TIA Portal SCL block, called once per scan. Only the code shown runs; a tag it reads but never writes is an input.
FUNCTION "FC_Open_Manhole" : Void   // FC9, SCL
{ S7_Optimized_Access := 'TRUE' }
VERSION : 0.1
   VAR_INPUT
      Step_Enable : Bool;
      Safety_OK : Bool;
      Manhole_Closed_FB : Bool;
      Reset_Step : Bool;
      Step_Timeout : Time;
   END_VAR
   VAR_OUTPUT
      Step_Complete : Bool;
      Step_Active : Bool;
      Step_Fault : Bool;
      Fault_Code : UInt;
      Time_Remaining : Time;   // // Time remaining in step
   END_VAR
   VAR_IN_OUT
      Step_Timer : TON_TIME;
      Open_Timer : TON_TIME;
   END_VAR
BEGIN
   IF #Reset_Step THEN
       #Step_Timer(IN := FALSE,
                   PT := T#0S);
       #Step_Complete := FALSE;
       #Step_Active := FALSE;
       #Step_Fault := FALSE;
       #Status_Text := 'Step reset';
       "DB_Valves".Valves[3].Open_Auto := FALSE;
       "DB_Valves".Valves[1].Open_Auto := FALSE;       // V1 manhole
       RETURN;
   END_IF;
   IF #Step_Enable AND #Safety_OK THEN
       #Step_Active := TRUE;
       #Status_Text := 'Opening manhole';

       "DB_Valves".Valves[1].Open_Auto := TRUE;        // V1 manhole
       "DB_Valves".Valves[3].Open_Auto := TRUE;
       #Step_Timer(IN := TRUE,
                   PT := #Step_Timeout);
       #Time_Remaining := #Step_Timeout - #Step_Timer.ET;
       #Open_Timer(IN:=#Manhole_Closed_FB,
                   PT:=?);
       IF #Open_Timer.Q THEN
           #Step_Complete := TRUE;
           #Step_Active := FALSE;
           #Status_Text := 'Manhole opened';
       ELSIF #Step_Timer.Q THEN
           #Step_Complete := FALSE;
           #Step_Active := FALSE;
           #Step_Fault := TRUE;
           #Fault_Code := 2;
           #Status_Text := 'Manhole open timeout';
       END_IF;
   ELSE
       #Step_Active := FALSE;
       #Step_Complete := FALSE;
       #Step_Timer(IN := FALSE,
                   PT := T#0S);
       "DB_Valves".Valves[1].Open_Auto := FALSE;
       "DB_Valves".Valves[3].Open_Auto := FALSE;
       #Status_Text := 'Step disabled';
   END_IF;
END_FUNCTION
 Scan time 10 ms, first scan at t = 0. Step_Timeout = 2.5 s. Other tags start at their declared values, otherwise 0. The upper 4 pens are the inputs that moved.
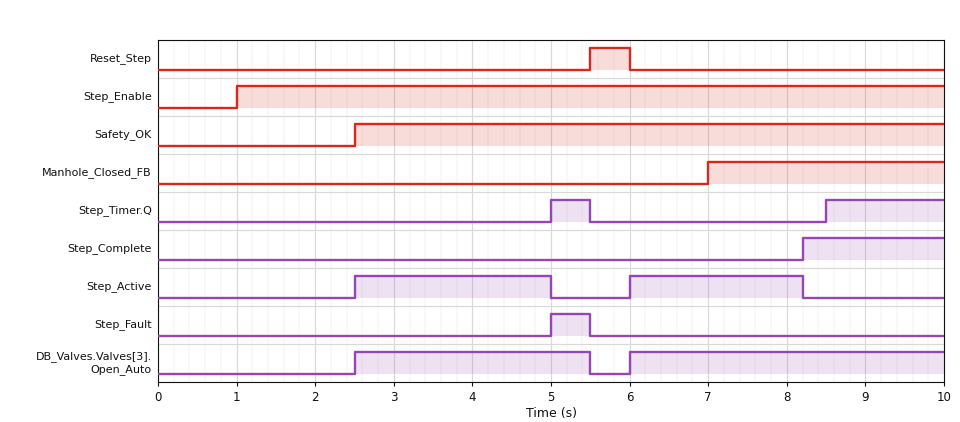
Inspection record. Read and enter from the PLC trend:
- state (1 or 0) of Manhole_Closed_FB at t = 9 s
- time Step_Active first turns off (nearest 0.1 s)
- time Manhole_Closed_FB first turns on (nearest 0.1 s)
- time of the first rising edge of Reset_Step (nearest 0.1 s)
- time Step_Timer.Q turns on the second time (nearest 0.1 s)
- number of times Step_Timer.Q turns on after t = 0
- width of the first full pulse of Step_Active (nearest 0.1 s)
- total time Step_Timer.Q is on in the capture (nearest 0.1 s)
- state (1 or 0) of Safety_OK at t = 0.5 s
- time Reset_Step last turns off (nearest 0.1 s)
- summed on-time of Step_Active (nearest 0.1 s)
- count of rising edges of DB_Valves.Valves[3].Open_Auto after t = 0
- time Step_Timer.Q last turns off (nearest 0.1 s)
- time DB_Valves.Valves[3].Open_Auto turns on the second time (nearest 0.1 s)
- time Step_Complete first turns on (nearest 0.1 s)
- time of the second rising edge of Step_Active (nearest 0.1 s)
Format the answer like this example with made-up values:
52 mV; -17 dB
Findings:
1; 5.0 s; 7.0 s; 5.5 s; 8.5 s; 2; 2.5 s; 2.0 s; 0; 6.0 s; 4.7 s; 2; 5.5 s; 6.0 s; 8.2 s; 6.0 s
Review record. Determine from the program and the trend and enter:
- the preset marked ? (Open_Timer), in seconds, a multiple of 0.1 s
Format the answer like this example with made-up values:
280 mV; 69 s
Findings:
1.2 s
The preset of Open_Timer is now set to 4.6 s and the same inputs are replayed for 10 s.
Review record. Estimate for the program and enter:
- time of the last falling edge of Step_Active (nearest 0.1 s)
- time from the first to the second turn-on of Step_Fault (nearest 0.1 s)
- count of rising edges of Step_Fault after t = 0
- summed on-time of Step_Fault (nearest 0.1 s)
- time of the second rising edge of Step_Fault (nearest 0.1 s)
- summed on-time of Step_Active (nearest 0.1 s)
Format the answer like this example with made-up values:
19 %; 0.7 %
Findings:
8.5 s; 3.5 s; 2; 2.0 s; 8.5 s; 5.0 s
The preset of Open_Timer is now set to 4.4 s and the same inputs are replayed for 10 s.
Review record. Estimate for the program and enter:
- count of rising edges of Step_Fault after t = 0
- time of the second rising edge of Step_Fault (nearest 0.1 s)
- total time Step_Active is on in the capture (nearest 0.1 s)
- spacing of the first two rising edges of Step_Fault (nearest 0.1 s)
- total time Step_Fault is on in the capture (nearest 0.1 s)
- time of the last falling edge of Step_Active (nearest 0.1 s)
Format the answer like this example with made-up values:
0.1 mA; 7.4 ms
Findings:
2; 8.5 s; 5.0 s; 3.5 s; 2.0 s; 8.5 s
